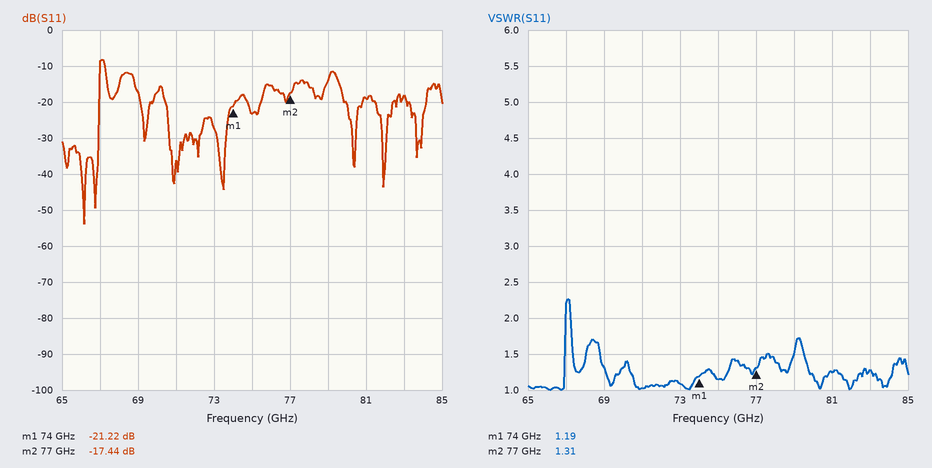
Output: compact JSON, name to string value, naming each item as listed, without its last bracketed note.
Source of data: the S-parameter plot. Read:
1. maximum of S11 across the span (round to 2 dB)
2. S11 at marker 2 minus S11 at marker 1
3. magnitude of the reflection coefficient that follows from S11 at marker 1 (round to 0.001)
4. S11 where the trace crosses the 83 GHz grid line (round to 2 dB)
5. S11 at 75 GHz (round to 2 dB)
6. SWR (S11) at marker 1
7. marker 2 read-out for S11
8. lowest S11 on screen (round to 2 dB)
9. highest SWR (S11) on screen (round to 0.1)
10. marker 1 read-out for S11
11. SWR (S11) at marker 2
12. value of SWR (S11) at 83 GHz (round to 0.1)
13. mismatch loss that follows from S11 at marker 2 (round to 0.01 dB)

{"maximum of S11 across the span": "-8 dB", "S11 at marker 2 minus S11 at marker 1": "3.78 dB", "magnitude of the reflection coefficient that follows from S11 at marker 1": "0.087", "S11 where the trace crosses the 83 GHz grid line": "-18 dB", "S11 at 75 GHz": "-24 dB", "SWR (S11) at marker 1": "1.19", "marker 2 read-out for S11": "-17.44 dB", "lowest S11 on screen": "-54 dB", "highest SWR (S11) on screen": "2.3", "marker 1 read-out for S11": "-21.22 dB", "SWR (S11) at marker 2": "1.31", "value of SWR (S11) at 83 GHz": "1.3", "mismatch loss that follows from S11 at marker 2": "0.08 dB"}
